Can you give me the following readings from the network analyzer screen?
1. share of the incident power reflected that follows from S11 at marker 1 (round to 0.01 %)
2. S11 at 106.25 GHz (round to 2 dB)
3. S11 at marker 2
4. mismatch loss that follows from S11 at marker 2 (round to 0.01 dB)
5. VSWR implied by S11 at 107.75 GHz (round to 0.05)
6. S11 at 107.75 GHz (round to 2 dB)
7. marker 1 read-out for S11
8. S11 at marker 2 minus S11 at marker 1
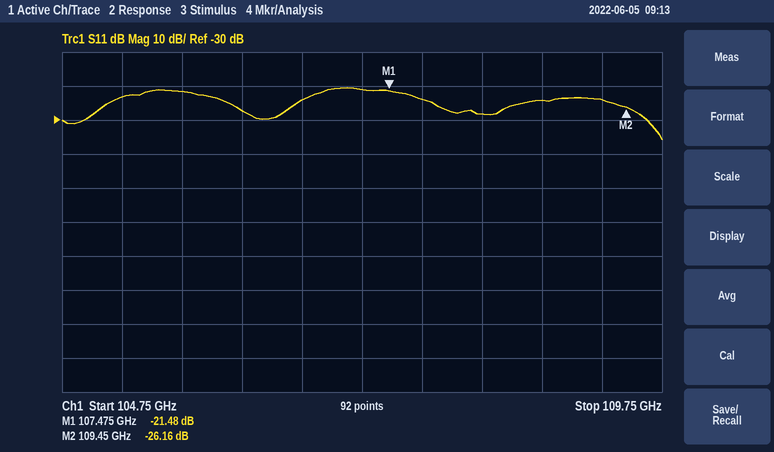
0.71 %
-28 dB
-26.16 dB
0.01 dB
1.15
-24 dB
-21.48 dB
-4.68 dB
